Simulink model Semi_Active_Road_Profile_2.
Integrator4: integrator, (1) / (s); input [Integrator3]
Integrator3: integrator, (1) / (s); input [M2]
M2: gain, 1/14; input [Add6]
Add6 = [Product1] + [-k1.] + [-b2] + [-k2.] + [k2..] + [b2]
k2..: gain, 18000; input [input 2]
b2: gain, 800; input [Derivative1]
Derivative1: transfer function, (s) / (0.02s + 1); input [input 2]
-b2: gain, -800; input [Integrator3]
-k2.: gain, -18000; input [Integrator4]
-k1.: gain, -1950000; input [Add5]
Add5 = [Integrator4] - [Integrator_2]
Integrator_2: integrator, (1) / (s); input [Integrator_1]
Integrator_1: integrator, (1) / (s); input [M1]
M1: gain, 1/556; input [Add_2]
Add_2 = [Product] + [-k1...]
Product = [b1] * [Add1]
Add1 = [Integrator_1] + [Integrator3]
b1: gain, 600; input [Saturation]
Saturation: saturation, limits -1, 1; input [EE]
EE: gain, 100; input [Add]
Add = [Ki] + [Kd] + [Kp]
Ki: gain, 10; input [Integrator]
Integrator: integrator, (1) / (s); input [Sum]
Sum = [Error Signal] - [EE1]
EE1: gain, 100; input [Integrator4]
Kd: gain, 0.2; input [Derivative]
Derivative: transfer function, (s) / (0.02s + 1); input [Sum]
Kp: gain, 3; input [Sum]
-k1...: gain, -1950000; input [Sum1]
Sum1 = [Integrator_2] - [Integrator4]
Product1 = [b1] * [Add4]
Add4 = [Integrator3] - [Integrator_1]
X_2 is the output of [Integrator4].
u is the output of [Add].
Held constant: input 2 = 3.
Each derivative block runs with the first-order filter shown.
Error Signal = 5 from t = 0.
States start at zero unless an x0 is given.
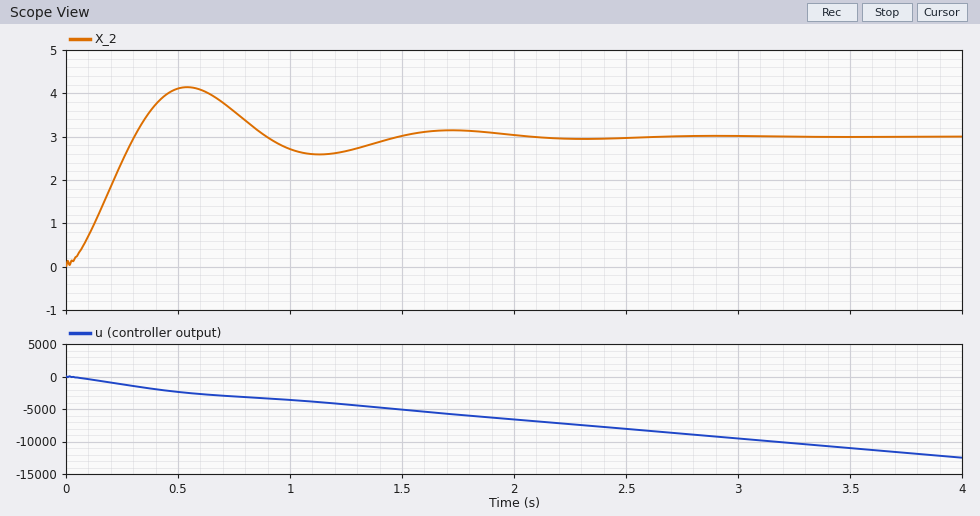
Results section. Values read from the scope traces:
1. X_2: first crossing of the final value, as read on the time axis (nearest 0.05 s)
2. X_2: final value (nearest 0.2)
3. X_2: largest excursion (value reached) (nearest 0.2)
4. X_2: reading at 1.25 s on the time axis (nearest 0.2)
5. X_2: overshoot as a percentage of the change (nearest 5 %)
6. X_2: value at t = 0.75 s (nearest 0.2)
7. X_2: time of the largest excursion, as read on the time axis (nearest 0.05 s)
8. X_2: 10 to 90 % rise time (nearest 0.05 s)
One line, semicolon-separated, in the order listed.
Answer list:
0.30 s; 3.0; 4.2; 2.6; 40 %; 3.6; 0.55 s; 0.20 s
